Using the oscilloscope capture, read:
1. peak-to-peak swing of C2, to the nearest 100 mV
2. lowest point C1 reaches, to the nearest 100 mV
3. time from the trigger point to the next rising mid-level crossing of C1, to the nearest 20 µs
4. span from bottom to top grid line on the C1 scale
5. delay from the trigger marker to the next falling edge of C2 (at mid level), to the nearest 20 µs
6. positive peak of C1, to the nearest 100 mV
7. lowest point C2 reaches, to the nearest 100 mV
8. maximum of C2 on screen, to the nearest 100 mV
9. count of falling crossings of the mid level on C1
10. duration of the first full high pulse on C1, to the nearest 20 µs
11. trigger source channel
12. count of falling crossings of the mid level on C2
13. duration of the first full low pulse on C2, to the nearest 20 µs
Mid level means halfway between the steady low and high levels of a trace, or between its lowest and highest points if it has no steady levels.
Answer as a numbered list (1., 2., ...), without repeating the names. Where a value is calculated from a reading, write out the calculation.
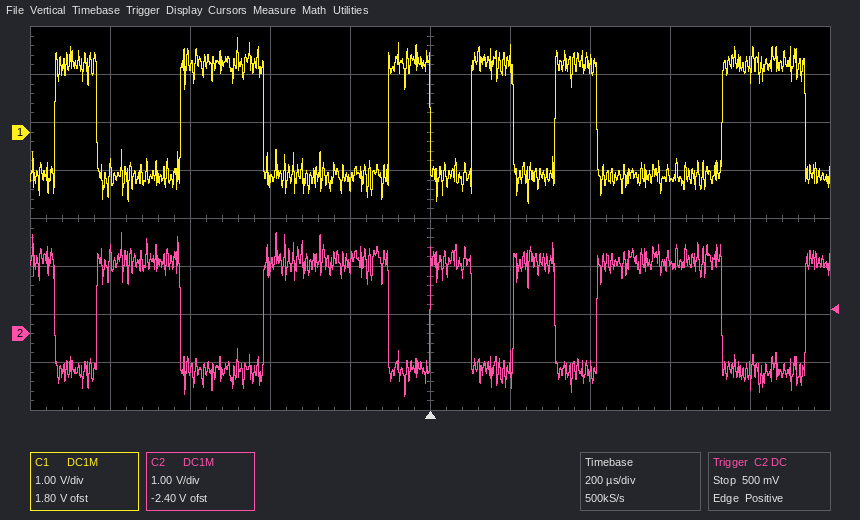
1. 2.1 V − (-1.3 V) = 3.4 V
2. -1.5 V
3. 100 µs
4. 8 V
5. 100 µs
6. 2.0 V
7. -1.3 V
8. 2.1 V
9. 6
10. 100 µs
11. C2
12. 6
13. 100 µs
